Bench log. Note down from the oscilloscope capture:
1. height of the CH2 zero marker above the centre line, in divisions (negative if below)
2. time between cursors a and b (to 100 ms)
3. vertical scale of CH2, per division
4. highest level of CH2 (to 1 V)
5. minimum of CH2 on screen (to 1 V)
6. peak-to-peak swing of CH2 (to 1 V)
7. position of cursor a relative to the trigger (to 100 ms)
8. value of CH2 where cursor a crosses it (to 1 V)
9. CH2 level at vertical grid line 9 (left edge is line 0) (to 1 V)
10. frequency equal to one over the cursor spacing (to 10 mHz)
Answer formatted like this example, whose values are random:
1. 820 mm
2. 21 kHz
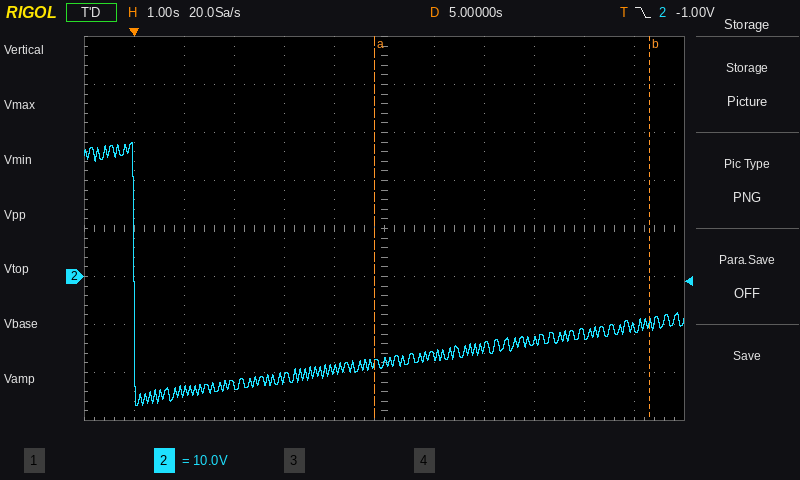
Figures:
1. -1.0 div
2. 5.5 s
3. 10 V
4. 28 V
5. -27 V
6. 55 V
7. +4.8 s
8. -18 V
9. -13 V
10. 180 mHz
